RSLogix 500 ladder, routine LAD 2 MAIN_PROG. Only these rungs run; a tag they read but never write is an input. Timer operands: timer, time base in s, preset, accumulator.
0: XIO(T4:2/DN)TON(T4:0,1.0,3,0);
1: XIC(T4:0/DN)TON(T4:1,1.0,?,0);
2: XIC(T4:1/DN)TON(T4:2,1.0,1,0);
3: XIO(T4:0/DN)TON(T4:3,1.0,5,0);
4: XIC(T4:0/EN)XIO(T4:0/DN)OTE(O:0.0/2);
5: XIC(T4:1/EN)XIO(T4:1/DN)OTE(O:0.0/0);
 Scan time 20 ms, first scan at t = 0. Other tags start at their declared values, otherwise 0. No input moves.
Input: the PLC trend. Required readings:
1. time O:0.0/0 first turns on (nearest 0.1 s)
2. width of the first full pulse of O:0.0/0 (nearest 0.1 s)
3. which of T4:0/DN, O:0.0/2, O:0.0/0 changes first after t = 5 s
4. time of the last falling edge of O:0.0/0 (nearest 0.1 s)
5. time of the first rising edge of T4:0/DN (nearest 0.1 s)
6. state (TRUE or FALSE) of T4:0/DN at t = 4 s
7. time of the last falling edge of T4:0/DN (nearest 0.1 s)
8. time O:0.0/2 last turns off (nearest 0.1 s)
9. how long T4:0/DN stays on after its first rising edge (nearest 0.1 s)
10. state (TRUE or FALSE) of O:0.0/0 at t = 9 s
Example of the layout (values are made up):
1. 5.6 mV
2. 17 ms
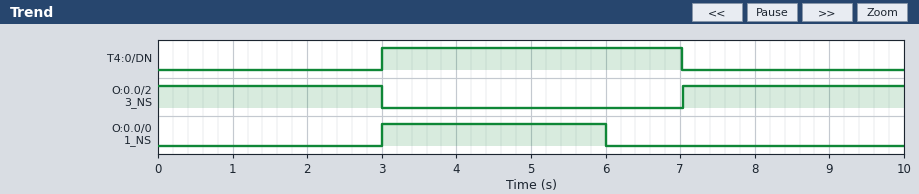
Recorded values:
1. 3.0 s
2. 3.0 s
3. O:0.0/0
4. 6.0 s
5. 3.0 s
6. TRUE
7. 7.0 s
8. 3.0 s
9. 4.0 s
10. FALSE
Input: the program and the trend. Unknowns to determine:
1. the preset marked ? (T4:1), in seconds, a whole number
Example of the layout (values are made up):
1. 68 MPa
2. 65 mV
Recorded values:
1. 3 s
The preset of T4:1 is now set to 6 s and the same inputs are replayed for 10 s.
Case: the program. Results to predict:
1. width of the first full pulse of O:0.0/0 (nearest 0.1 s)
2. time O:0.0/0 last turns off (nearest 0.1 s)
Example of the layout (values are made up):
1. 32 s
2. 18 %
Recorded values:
1. 6.0 s
2. 9.0 s
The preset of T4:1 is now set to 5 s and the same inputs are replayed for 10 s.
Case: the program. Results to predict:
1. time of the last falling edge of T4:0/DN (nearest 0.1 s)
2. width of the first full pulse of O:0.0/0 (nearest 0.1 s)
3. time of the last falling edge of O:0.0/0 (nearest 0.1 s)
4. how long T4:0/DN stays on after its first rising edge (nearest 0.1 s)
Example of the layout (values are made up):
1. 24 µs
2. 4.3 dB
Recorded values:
1. 9.0 s
2. 5.0 s
3. 8.0 s
4. 6.0 s
